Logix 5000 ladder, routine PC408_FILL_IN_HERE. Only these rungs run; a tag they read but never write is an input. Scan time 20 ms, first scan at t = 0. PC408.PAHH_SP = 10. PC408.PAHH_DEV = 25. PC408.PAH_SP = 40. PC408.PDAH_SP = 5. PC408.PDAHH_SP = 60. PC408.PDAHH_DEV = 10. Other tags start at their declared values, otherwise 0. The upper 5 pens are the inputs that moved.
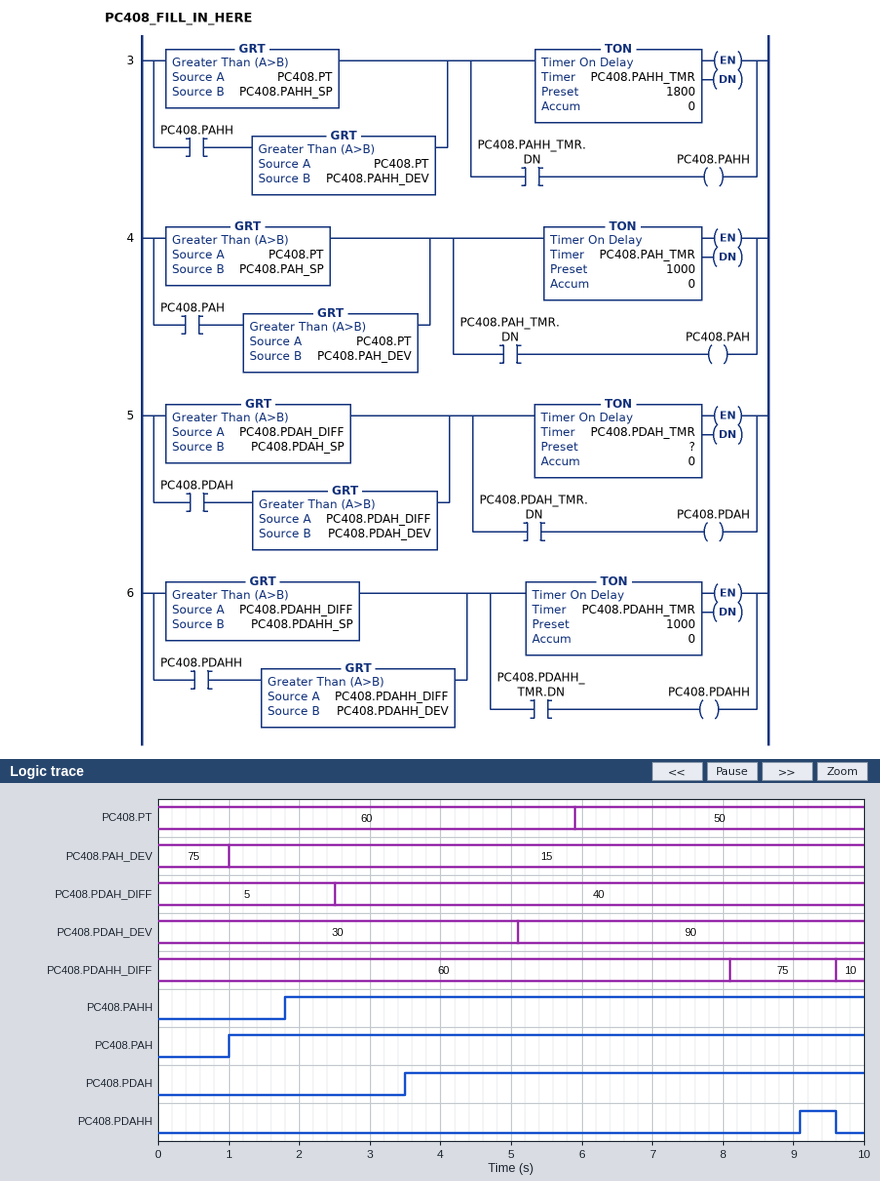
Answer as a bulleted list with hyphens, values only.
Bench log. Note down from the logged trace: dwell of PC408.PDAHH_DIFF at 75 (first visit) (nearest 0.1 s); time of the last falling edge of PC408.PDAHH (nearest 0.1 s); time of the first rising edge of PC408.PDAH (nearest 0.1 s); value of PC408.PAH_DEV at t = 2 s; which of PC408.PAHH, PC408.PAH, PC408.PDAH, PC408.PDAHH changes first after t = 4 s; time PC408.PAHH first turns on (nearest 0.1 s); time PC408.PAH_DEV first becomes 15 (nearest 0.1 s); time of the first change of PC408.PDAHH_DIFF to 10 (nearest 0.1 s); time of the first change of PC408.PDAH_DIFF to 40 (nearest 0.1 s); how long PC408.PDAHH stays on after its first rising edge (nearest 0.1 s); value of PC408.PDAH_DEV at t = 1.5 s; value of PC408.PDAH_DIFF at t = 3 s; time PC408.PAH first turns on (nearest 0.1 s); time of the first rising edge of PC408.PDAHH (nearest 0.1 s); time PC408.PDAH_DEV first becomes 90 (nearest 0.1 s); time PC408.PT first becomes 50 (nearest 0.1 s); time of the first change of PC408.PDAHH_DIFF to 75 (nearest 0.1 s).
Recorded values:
- 1.5 s
- 9.6 s
- 3.5 s
- 15
- PC408.PDAHH
- 1.8 s
- 1.0 s
- 9.6 s
- 2.5 s
- 0.5 s
- 30
- 40
- 1.0 s
- 9.1 s
- 5.1 s
- 5.9 s
- 8.1 s
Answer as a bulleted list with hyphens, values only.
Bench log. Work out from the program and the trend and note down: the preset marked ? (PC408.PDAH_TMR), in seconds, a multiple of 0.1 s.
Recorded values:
- 1.0 s
